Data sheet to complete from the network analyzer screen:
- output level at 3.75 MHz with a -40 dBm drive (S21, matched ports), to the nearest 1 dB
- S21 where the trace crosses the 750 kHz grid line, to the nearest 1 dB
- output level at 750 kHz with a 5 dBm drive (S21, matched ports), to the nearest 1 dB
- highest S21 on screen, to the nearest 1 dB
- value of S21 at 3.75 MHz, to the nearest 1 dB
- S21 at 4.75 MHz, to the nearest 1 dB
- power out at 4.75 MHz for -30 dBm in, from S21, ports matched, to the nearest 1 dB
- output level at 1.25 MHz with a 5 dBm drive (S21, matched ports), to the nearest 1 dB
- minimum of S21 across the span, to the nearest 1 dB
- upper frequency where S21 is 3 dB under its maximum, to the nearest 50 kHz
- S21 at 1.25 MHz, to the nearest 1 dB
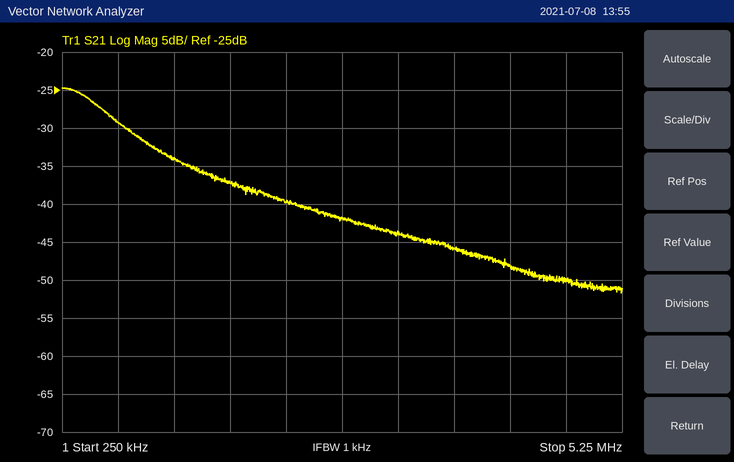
-86 dBm
-29 dB
-24 dBm
-25 dB
-46 dB
-50 dB
-80 dBm
-29 dBm
-52 dB
600 kHz
-34 dB
